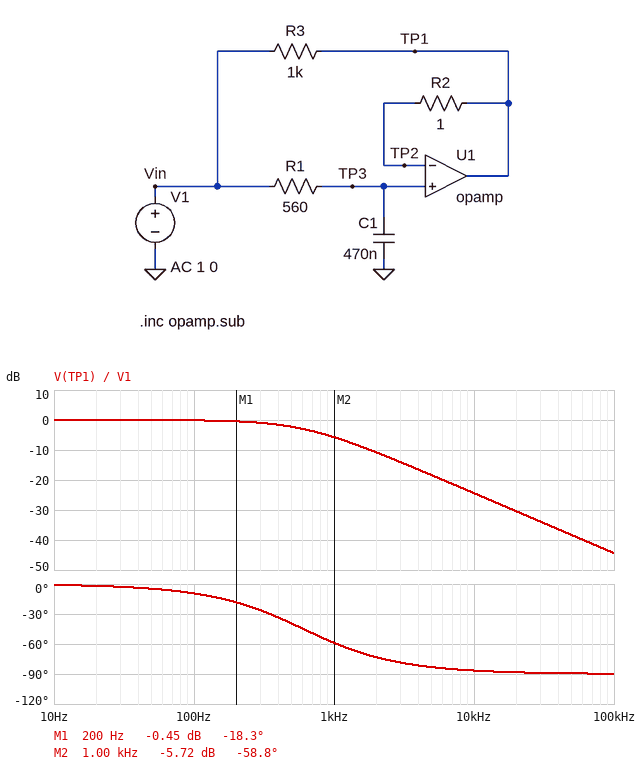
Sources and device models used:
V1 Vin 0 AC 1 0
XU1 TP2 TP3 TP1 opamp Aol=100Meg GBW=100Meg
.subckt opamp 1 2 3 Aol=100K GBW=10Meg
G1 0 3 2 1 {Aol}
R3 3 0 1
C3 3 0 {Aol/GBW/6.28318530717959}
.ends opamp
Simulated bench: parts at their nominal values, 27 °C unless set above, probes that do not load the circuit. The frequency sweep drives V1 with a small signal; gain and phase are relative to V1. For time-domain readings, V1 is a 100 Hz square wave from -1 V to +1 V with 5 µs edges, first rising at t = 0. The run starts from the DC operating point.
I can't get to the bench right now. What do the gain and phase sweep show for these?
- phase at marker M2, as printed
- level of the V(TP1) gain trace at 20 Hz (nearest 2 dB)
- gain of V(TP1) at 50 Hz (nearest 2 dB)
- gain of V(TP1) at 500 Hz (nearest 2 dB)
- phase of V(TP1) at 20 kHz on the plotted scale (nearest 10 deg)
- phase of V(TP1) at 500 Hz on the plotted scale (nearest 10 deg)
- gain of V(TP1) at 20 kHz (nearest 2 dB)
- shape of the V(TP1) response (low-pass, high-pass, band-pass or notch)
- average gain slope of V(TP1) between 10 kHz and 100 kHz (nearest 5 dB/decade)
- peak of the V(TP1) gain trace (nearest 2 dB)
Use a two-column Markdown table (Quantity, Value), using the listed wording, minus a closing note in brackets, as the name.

| Quantity | Value |
|---|---|
| phase at marker M2, as printed | -58.8 deg |
| level of the V(TP1) gain trace at 20 Hz | 0 dB |
| gain of V(TP1) at 50 Hz | 0 dB |
| gain of V(TP1) at 500 Hz | -2 dB |
| phase of V(TP1) at 20 kHz on the plotted scale | -90 deg |
| phase of V(TP1) at 500 Hz on the plotted scale | -40 deg |
| gain of V(TP1) at 20 kHz | -30 dB |
| shape of the V(TP1) response | low-pass |
| average gain slope of V(TP1) between 10 kHz and 100 kHz | -20 dB/decade |
| peak of the V(TP1) gain trace | 0 dB |
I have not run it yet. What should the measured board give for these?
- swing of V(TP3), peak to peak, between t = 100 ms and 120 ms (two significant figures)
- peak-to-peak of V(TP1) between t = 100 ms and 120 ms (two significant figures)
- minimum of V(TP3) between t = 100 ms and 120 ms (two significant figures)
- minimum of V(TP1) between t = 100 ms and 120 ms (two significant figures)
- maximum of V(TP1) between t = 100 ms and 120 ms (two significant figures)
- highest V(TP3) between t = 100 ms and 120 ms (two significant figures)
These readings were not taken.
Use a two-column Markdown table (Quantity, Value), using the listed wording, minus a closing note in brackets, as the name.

| Quantity | Value |
|---|---|
| swing of V(TP3), peak to peak, between t = 100 ms and 120 ms | 2.0 V |
| peak-to-peak of V(TP1) between t = 100 ms and 120 ms | 2.0 V |
| minimum of V(TP3) between t = 100 ms and 120 ms | -1.0 V |
| minimum of V(TP1) between t = 100 ms and 120 ms | -1.0 V |
| maximum of V(TP1) between t = 100 ms and 120 ms | 1.0 V |
| highest V(TP3) between t = 100 ms and 120 ms | 1.0 V |
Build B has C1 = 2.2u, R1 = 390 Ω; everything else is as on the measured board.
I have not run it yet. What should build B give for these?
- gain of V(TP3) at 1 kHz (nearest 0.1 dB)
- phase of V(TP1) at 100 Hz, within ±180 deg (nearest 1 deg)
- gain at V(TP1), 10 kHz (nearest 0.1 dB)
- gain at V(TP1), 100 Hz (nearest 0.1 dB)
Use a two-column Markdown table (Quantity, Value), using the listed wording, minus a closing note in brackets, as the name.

| Quantity | Value |
|---|---|
| gain of V(TP3) at 1 kHz | -14.8 dB |
| phase of V(TP1) at 100 Hz, within ±180 deg | -28 deg |
| gain at V(TP1), 10 kHz | -34.6 dB |
| gain at V(TP1), 100 Hz | -1.1 dB |
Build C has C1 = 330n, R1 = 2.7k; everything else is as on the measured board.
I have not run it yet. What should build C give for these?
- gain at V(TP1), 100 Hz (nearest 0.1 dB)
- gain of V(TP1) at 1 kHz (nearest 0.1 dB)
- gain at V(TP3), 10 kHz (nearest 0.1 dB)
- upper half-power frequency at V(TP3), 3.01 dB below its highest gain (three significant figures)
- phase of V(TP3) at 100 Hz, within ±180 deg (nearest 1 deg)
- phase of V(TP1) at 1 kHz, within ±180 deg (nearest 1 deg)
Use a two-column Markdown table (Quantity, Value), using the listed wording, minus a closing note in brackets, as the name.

| Quantity | Value |
|---|---|
| gain at V(TP1), 100 Hz | -1.2 dB |
| gain of V(TP1) at 1 kHz | -15.1 dB |
| gain at V(TP3), 10 kHz | -35.0 dB |
| upper half-power frequency at V(TP3), 3.01 dB below its highest gain | 179 Hz |
| phase of V(TP3) at 100 Hz, within ±180 deg | -29 deg |
| phase of V(TP1) at 1 kHz, within ±180 deg | -80 deg |
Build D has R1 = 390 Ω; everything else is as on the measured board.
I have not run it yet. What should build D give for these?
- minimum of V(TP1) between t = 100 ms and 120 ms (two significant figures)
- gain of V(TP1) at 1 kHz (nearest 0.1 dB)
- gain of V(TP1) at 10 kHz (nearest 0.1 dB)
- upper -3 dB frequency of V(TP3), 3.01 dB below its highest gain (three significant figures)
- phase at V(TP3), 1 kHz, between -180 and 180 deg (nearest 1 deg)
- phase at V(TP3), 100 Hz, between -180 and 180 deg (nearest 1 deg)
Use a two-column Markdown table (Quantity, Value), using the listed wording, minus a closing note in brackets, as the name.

| Quantity | Value |
|---|---|
| minimum of V(TP1) between t = 100 ms and 120 ms | -1.0 V |
| gain of V(TP1) at 1 kHz | -3.7 dB |
| gain of V(TP1) at 10 kHz | -21.3 dB |
| upper -3 dB frequency of V(TP3), 3.01 dB below its highest gain | 868 Hz |
| phase at V(TP3), 1 kHz, between -180 and 180 deg | -49 deg |
| phase at V(TP3), 100 Hz, between -180 and 180 deg | -7 deg |
